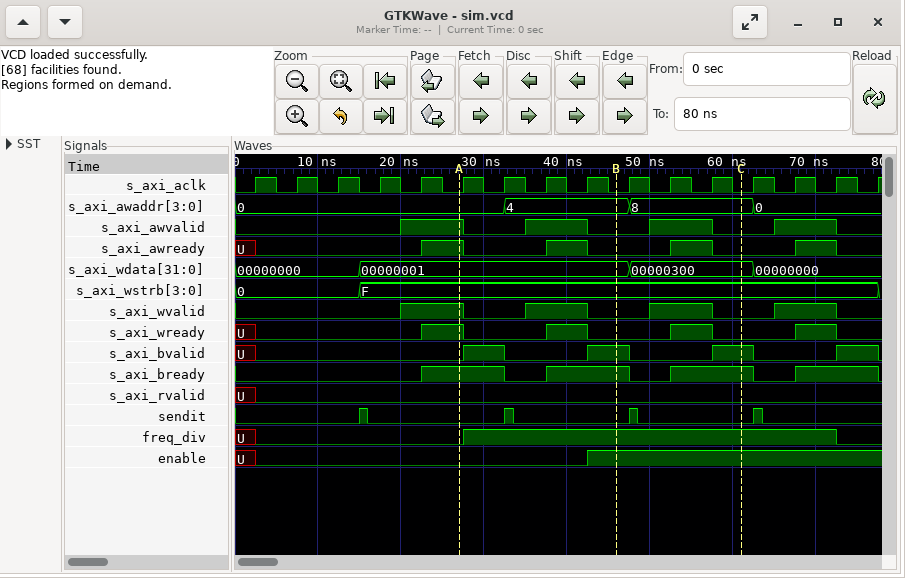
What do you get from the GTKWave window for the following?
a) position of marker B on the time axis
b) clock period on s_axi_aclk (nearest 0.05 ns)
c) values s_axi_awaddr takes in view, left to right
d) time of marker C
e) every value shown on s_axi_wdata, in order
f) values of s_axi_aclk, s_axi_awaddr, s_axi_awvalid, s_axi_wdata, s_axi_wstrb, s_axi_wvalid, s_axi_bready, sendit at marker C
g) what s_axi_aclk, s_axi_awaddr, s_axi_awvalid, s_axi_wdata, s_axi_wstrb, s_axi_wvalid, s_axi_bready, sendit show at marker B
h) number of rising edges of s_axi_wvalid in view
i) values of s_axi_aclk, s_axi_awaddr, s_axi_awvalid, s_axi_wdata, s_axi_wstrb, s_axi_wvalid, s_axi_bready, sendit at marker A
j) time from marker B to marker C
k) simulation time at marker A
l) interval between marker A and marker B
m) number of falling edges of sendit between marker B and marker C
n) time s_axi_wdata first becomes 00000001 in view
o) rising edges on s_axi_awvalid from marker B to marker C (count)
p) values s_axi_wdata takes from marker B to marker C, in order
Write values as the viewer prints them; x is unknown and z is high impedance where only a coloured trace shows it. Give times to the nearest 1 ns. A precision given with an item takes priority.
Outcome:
46 ns
5 ns
0, 4, 8, 0
61 ns
00000000, 00000001, 00000300, 00000000
s_axi_aclk=0, s_axi_awaddr=8, s_axi_awvalid=0, s_axi_wdata=00000300, s_axi_wstrb=F, s_axi_wvalid=0, s_axi_bready=1, sendit=0
s_axi_aclk=0, s_axi_awaddr=4, s_axi_awvalid=0, s_axi_wdata=00000001, s_axi_wstrb=F, s_axi_wvalid=0, s_axi_bready=1, sendit=0
4
s_axi_aclk=0, s_axi_awaddr=0, s_axi_awvalid=1, s_axi_wdata=00000001, s_axi_wstrb=F, s_axi_wvalid=1, s_axi_bready=1, sendit=0
15 ns
27 ns
19 ns
1
15 ns
1
00000001, 00000300
